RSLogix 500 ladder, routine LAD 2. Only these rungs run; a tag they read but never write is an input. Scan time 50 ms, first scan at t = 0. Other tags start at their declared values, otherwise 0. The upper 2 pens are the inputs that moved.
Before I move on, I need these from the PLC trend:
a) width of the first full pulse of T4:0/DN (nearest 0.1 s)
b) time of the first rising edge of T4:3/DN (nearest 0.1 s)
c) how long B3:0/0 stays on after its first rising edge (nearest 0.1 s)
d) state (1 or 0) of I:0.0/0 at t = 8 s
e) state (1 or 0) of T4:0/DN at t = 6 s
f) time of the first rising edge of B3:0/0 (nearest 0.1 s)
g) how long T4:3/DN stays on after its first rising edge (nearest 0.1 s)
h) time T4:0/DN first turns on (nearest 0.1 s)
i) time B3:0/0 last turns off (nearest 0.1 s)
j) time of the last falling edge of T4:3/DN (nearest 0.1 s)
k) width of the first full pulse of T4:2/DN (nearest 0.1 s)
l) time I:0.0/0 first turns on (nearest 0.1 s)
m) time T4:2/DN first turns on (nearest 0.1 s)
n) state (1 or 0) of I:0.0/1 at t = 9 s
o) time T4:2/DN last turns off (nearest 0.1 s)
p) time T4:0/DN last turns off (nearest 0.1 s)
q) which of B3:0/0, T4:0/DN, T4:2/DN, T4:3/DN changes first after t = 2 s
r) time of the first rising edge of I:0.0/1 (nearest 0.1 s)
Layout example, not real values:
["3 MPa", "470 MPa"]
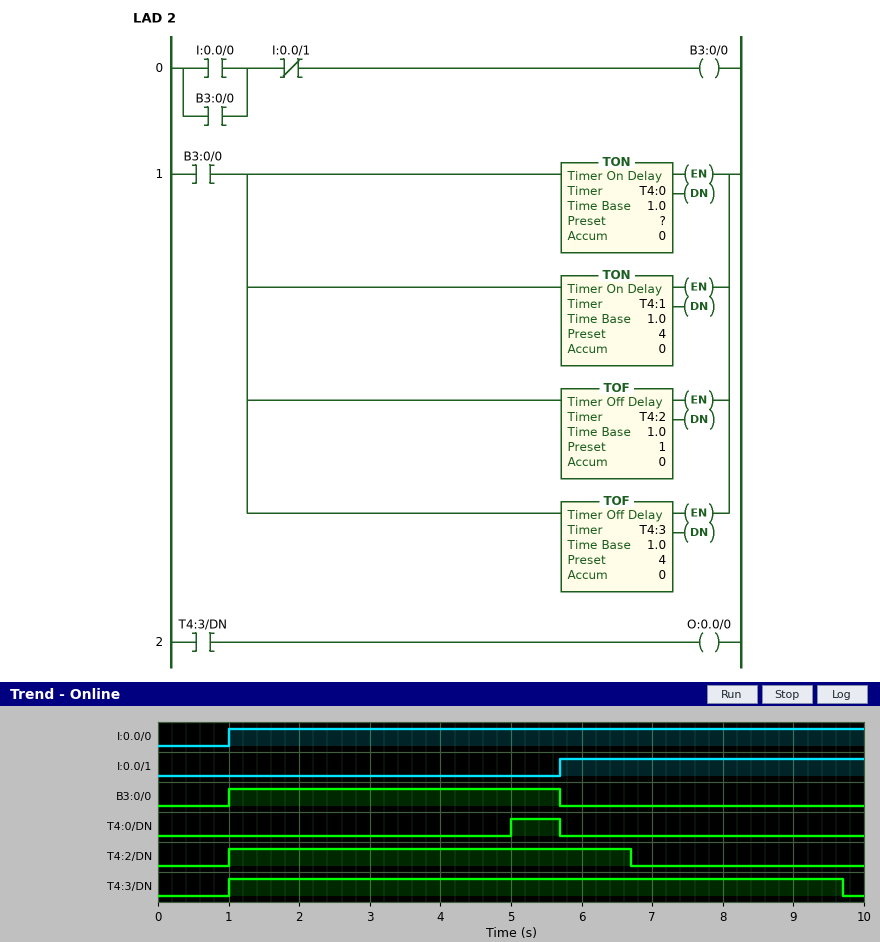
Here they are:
["0.7 s", "1.0 s", "4.7 s", "1", "0", "1.0 s", "8.7 s", "5.0 s", "5.7 s", "9.7 s", "5.7 s", "1.0 s", "1.0 s", "1", "6.7 s", "5.7 s", "T4:0/DN", "5.7 s"]
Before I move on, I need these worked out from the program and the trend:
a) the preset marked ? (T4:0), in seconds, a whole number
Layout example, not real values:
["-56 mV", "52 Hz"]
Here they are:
["4 s"]
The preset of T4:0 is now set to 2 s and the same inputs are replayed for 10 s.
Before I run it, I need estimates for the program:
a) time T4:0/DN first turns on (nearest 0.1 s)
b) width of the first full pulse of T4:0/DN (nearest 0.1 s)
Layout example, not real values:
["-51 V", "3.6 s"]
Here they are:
["3.0 s", "2.7 s"]
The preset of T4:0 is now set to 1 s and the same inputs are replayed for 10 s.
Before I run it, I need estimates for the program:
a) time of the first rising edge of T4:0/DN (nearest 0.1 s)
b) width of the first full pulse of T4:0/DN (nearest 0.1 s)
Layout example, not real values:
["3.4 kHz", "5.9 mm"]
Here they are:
["2.0 s", "3.7 s"]
